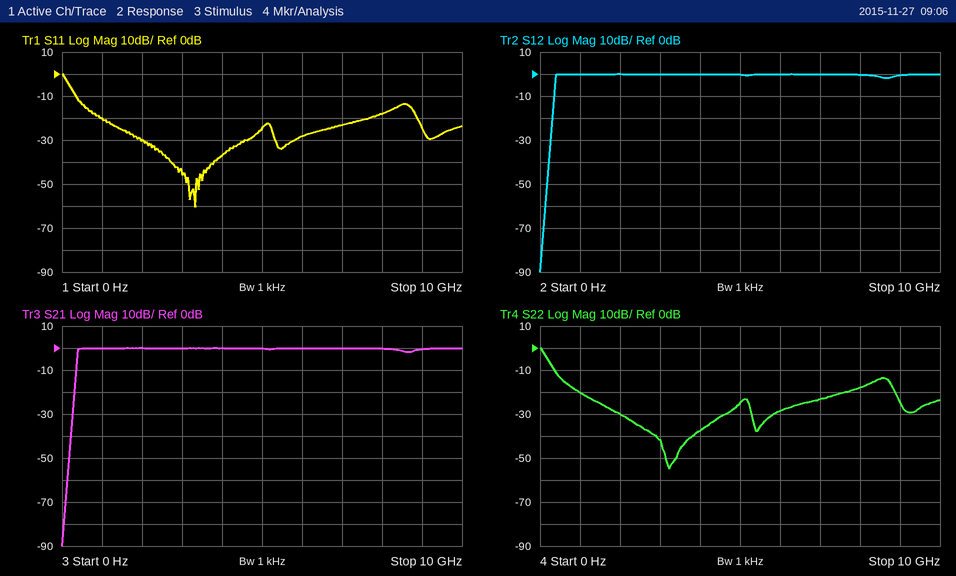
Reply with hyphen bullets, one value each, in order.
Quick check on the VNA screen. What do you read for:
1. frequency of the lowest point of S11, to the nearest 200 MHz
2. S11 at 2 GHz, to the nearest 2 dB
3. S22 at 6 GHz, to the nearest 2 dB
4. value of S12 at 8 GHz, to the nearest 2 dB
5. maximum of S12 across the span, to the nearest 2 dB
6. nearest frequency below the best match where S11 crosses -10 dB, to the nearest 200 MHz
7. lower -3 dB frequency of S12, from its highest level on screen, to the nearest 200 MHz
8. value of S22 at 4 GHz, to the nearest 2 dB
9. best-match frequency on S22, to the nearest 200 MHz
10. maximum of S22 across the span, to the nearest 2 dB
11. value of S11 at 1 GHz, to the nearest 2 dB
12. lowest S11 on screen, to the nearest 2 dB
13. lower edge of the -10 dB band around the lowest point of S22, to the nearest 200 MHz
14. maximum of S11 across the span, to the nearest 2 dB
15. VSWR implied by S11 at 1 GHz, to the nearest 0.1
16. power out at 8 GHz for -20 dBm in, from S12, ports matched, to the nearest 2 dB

- 3.4 GHz
- -30 dB
- -28 dB
- 0 dB
- 0 dB
- 400 MHz
- 400 MHz
- -38 dB
- 3.2 GHz
- 0 dB
- -20 dB
- -60 dB
- 400 MHz
- 0 dB
- 1.2
- -20 dBm
